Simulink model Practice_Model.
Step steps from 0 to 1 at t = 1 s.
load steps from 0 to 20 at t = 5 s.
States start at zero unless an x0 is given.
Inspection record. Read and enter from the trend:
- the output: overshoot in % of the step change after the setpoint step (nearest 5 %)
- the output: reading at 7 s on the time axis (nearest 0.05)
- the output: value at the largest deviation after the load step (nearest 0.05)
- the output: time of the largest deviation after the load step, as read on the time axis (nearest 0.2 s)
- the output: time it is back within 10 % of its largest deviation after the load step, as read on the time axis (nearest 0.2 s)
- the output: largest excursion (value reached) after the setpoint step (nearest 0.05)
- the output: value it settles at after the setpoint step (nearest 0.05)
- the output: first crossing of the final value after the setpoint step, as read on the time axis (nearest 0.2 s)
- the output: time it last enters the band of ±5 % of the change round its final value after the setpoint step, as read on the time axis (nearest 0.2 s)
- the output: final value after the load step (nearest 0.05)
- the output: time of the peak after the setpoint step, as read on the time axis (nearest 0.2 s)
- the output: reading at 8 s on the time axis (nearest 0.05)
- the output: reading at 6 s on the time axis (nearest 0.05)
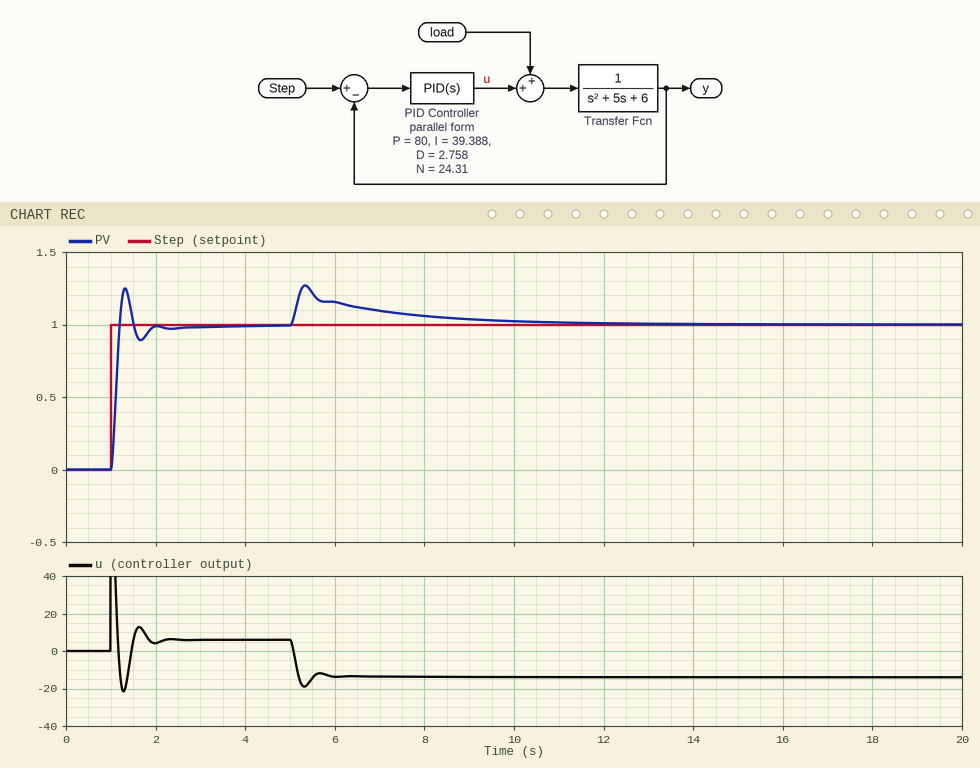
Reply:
25 %
1.10
1.25
5.4 s
9.6 s
1.25
1.00
1.2 s
1.8 s
1.00
1.4 s
1.05
1.15
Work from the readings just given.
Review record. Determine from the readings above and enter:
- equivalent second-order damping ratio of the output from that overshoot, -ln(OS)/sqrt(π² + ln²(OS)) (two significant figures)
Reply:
0.40
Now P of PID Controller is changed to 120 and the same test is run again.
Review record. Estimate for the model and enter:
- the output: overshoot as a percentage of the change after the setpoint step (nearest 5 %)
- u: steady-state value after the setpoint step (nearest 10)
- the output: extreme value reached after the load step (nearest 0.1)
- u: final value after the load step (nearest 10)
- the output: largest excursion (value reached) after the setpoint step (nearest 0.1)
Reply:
35 %
10
1.2
-10
1.3
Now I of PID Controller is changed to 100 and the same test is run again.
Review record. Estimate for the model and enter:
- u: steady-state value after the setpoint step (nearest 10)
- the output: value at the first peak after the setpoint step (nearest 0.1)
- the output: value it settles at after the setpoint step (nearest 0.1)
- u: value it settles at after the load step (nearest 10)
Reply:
10
1.3
1.0
-10
